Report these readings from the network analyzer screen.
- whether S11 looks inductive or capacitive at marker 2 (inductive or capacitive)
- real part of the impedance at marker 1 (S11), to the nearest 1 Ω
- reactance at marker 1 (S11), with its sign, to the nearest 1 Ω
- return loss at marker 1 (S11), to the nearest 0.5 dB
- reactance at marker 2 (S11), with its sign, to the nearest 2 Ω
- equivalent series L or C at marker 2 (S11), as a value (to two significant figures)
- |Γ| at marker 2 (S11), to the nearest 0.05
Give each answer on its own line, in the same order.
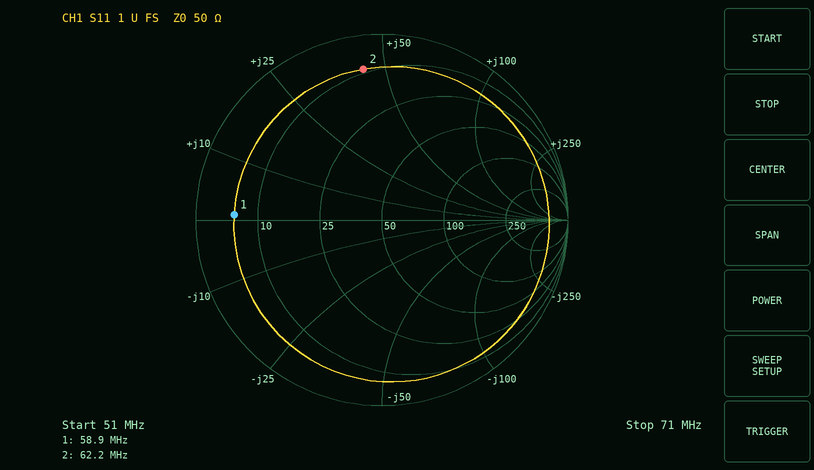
inductive
6 Ω
+1 Ω
2.0 dB
+44 Ω
110 nH
0.80
